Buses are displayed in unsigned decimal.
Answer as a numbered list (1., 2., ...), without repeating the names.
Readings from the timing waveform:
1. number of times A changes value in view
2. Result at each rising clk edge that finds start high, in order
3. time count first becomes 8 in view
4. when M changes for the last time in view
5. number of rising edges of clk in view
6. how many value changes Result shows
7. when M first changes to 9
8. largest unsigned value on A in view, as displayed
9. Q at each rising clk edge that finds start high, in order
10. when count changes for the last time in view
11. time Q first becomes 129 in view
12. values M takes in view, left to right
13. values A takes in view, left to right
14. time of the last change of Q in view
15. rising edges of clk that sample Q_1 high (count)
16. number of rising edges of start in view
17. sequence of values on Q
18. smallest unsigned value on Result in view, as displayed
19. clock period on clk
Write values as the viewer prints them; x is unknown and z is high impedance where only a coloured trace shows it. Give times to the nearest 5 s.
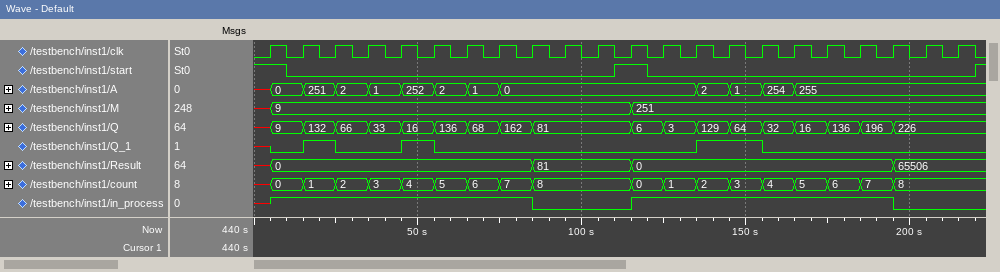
1. 12
2. x, 81
3. 85 s
4. 115 s
5. 22
6. 4
7. 5 s
8. 255
9. x, 81
10. 195 s
11. 135 s
12. x, 9, 251
13. x, 0, 251, 2, 1, 252, 2, 1, 0, 2, 1, 254, 255
14. 195 s
15. 4
16. 2
17. x, 9, 132, 66, 33, 16, 136, 68, 162, 81, 6, 3, 129, 64, 32, 16, 136, 196, 226
18. 0
19. 10 s
